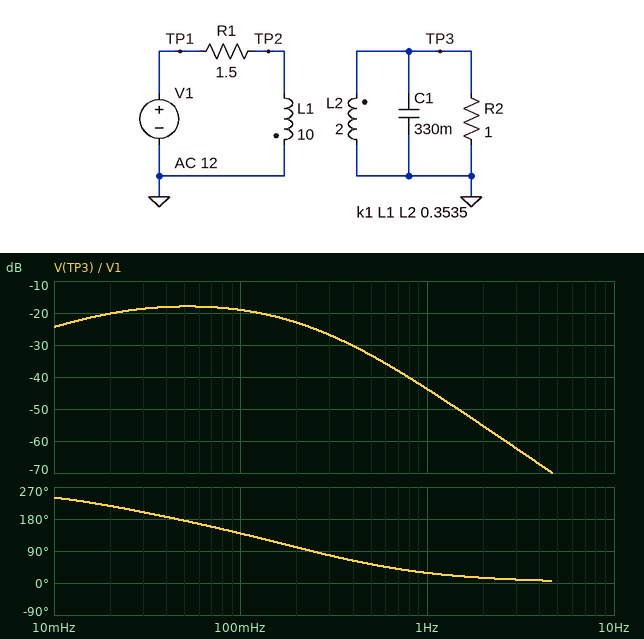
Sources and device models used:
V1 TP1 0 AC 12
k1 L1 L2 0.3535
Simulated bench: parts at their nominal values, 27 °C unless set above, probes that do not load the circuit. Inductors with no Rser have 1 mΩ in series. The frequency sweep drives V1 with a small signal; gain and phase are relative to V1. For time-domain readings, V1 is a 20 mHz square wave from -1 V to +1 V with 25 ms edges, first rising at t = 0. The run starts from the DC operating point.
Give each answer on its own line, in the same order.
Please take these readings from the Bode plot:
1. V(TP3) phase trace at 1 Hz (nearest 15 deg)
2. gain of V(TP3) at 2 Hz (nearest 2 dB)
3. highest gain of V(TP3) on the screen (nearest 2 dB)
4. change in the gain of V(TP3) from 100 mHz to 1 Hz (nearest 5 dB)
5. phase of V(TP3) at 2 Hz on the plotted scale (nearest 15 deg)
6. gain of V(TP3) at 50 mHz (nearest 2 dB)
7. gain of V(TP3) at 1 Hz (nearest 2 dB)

30 deg
-56 dB
-18 dB
-25 dB
15 deg
-18 dB
-44 dB
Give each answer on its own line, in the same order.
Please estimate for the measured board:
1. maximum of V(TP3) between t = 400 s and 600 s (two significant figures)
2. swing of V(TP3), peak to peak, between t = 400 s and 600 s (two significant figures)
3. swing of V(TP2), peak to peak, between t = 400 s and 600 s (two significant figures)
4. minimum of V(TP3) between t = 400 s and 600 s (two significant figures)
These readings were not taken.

200 mV
400 mV
3.9 V
-200 mV
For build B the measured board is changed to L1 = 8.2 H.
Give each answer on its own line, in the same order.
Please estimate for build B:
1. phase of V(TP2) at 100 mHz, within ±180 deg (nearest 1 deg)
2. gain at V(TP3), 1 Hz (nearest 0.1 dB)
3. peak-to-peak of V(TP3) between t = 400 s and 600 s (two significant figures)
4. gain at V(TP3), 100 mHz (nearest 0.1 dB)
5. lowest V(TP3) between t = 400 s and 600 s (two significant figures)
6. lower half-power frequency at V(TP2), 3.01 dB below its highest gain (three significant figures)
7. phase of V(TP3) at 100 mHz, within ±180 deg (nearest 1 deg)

17 deg
-42.9 dB
420 mV
-18.3 dB
-210 mV
30.9 mHz
142 deg
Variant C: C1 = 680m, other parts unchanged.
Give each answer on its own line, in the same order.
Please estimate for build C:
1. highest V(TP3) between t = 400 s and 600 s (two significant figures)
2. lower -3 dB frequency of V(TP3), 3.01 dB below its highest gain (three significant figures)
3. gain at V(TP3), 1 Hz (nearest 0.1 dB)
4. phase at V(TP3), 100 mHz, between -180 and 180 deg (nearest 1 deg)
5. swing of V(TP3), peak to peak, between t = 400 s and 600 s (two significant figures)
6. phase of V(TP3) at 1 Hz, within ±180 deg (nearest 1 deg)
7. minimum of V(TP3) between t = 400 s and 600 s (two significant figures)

210 mV
18.5 mHz
-49.5 dB
130 deg
420 mV
15 deg
-210 mV
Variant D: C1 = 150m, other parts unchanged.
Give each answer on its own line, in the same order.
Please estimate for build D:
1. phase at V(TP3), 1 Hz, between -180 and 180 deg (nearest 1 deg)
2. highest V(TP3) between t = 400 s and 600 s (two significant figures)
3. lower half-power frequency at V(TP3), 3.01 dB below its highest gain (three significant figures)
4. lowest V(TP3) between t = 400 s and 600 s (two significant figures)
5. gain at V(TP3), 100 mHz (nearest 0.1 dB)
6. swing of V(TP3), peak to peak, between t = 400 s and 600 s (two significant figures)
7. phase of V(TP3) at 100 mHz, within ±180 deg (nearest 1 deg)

51 deg
190 mV
16.6 mHz
-190 mV
-19.5 dB
380 mV
143 deg
